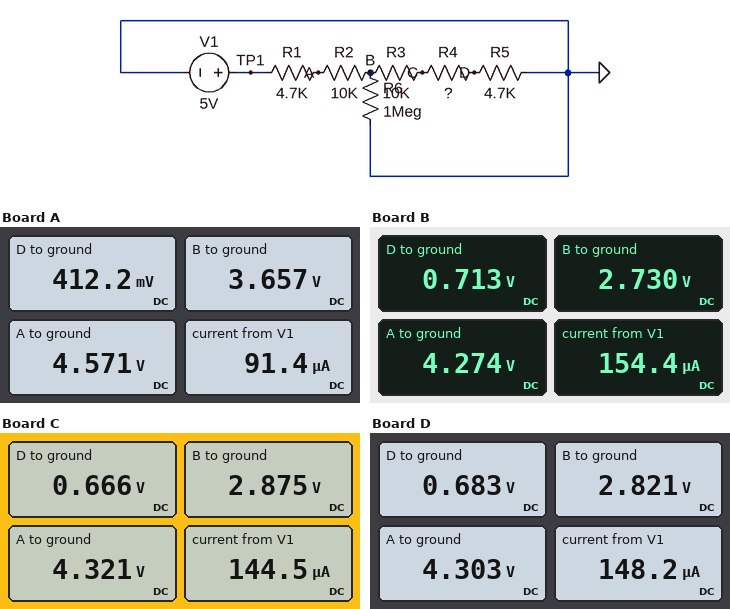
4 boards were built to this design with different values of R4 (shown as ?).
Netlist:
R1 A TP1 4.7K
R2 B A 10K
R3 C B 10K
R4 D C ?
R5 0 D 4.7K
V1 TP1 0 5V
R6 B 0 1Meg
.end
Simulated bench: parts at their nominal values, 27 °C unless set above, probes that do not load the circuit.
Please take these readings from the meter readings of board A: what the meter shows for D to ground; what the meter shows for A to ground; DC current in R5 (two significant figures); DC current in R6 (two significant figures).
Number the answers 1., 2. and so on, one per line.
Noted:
1. 412.2 mV
2. 4.571 V
3. 88 µA
4. 3.7 µA
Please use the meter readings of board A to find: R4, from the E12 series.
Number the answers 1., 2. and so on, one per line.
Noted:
1. 27 kΩ
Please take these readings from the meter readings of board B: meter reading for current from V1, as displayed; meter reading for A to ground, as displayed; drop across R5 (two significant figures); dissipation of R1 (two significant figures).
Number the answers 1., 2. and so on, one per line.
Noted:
1. 154.4 µA
2. 4.274 V
3. 710 mV
4. 110 µW
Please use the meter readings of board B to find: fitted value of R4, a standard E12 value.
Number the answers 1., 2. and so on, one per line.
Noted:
1. 3.3 kΩ
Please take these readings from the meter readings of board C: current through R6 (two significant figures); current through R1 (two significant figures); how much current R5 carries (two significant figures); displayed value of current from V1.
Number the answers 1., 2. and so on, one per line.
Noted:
1. 2.9 µA
2. 140 µA
3. 140 µA
4. 144.5 µA
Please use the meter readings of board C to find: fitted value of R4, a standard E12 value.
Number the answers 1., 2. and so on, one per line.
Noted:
1. 5.6 kΩ
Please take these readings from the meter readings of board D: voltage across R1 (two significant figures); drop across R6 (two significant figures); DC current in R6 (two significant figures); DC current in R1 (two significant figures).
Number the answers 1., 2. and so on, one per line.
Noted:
1. 700 mV
2. 2.8 V
3. 2.8 µA
4. 150 µA
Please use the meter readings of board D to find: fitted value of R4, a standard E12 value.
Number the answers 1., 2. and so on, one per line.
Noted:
1. 4.7 kΩ
